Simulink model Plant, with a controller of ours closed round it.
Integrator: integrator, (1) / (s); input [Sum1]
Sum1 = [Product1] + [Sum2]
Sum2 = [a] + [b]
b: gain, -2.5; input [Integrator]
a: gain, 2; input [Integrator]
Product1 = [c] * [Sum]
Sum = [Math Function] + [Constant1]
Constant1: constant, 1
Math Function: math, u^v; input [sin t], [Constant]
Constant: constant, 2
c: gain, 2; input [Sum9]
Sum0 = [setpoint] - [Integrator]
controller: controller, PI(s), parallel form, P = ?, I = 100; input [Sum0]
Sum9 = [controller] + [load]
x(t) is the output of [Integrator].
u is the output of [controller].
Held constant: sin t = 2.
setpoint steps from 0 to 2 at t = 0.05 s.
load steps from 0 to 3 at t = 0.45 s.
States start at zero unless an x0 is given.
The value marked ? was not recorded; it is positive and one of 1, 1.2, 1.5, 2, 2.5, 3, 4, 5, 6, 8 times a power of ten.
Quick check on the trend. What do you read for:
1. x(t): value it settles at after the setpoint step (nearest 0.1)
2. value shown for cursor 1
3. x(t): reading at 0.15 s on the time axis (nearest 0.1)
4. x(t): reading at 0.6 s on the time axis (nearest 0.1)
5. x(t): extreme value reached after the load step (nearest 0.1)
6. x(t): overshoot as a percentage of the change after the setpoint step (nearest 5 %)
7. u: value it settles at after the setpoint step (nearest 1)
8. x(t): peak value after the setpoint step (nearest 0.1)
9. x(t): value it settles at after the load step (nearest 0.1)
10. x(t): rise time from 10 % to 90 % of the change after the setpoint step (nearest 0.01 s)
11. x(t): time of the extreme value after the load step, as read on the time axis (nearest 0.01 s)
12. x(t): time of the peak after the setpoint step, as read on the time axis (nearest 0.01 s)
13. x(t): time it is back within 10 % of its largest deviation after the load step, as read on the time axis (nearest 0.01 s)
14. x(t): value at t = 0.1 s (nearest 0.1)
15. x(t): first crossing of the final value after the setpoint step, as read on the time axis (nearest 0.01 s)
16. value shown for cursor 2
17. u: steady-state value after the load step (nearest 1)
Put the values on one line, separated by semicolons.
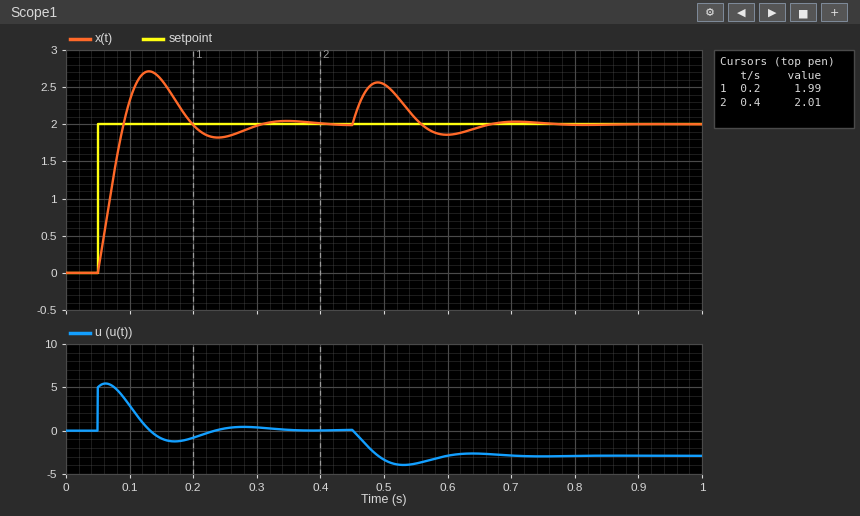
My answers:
2.0; 1.99; 2.6; 1.9; 2.6; 35 %; 0; 2.7; 2.0; 0.03 s; 0.49 s; 0.13 s; 0.64 s; 2.3; 0.09 s; 2.01; -3
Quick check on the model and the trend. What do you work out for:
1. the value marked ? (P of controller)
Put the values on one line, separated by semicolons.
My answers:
2.5
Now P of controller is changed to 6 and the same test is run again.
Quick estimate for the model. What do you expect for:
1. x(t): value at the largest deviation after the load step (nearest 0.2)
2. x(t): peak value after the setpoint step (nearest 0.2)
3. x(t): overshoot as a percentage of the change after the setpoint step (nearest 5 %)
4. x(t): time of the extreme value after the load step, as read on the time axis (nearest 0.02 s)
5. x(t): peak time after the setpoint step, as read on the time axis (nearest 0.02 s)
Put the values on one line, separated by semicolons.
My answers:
2.4; 2.2; 15 %; 0.48 s; 0.12 s
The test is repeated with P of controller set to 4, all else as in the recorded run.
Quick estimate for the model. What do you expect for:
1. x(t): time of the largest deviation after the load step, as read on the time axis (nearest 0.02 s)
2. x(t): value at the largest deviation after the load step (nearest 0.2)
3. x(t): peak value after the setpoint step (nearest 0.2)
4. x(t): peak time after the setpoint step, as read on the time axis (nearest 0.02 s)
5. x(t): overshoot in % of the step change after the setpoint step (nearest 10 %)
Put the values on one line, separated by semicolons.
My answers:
0.48 s; 2.4; 2.4; 0.12 s; 20 %
